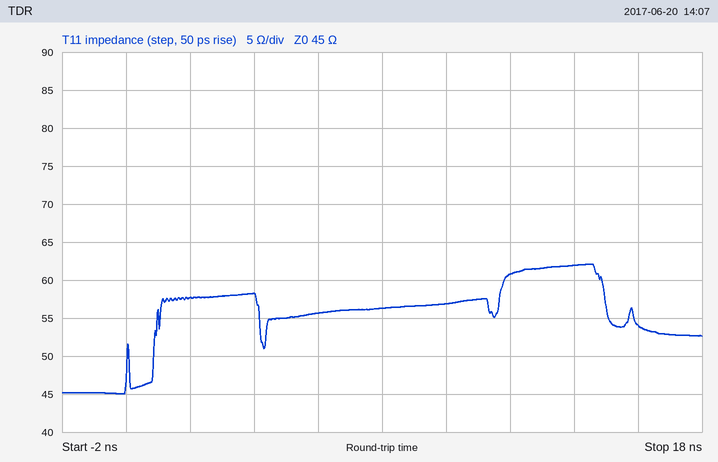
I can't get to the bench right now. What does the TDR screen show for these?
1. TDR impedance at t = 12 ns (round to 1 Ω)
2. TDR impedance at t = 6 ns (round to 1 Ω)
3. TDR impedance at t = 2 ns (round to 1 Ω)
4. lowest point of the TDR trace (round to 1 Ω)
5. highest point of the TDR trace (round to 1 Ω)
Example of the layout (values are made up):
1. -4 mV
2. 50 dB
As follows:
1. 61 Ω
2. 56 Ω
3. 58 Ω
4. 45 Ω
5. 62 Ω
